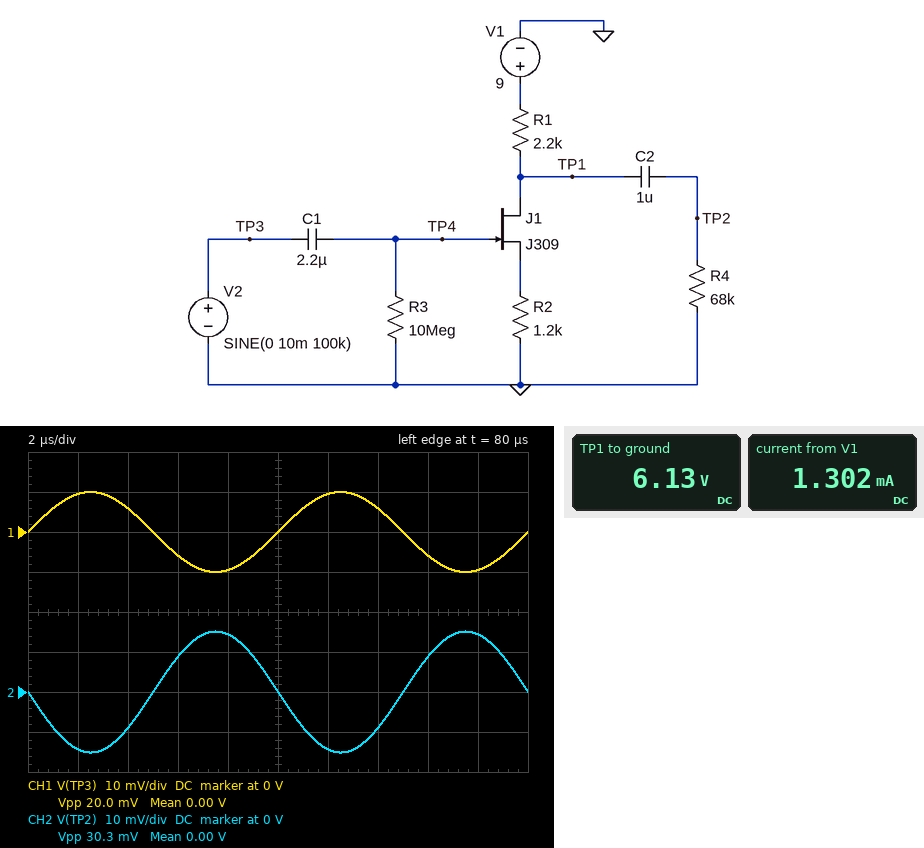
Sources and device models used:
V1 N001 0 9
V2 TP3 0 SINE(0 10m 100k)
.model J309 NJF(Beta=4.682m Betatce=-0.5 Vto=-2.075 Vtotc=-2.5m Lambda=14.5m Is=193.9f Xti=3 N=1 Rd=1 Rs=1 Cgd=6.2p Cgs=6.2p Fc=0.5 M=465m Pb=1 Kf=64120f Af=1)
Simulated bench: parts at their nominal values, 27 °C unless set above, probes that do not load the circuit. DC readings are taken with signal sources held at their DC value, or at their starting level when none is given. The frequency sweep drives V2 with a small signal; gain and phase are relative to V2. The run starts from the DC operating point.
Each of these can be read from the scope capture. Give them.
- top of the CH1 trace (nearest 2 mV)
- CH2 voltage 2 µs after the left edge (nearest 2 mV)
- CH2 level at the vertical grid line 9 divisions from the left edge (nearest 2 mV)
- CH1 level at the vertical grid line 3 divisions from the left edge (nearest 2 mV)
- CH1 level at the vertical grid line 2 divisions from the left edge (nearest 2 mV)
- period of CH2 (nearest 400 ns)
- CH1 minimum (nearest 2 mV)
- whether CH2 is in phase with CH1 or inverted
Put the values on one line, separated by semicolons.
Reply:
10 mV; -14 mV; 14 mV; -6 mV; 6 mV; 10.0 µs; -10 mV; inverted
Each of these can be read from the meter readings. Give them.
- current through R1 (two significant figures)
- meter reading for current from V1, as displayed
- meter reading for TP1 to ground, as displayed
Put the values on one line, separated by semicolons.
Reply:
1.3 mA; 1.302 mA; 6.13 V
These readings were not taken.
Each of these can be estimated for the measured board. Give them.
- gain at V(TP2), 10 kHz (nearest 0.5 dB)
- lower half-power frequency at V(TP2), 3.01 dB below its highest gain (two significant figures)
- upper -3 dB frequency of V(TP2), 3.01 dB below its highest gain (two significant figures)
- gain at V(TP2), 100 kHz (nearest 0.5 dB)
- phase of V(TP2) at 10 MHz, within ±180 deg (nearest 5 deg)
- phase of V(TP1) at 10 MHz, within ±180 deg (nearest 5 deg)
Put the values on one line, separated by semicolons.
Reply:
3.5 dB; 2.3 Hz; 320 MHz; 3.5 dB; 150 deg; 150 deg
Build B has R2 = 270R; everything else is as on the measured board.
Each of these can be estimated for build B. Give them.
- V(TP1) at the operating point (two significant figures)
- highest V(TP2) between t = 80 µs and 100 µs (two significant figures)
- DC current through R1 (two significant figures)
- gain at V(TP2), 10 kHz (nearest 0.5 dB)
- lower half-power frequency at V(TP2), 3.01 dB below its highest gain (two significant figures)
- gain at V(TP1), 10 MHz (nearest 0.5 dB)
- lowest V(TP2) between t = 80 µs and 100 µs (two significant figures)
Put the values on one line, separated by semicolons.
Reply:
1.3 V; 4.3 mV; 3.5 mA; -7.5 dB; 48 MHz; -7.0 dB; -4.2 mV
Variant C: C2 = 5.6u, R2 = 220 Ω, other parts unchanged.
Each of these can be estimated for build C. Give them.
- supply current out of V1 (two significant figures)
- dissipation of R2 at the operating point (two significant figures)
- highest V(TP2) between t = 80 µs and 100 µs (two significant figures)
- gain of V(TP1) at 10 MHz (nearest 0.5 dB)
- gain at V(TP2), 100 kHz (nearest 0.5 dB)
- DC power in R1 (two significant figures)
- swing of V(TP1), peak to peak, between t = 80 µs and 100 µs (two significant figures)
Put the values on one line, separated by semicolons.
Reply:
3.6 mA; 2.8 mW; 3.0 mV; -9.5 dB; -10.5 dB; 28 mW; 6.0 mV
